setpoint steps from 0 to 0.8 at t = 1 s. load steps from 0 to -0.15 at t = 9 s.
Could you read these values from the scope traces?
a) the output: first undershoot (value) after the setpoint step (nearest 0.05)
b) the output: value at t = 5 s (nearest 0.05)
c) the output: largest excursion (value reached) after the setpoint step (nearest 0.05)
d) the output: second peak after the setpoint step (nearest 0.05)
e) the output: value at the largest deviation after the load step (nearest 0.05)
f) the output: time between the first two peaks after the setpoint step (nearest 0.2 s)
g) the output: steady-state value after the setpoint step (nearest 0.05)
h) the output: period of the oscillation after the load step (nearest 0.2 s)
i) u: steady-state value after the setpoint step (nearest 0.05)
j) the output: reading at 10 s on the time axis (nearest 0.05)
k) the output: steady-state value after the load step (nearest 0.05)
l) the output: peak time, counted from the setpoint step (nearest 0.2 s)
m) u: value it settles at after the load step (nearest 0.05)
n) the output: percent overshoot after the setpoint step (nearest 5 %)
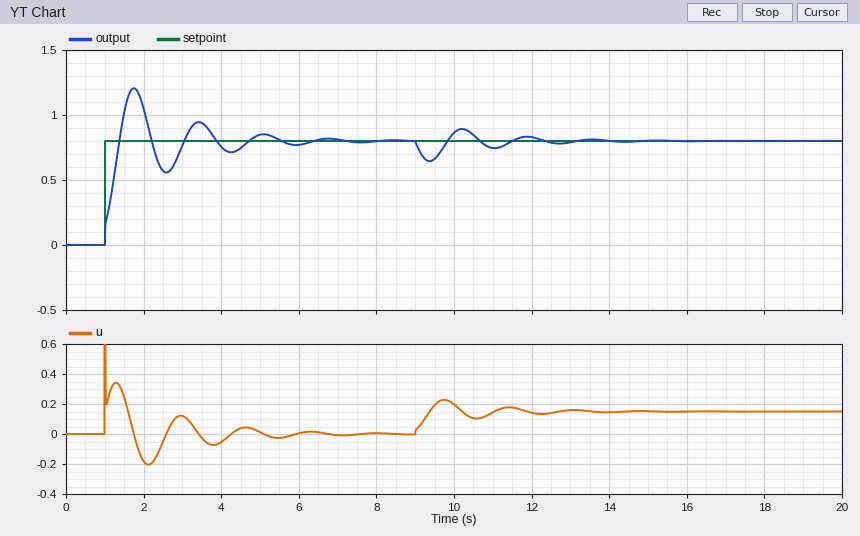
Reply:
0.55
0.85
1.20
0.95
0.65
1.6 s
0.80
1.6 s
0.00
0.85
0.80
0.8 s
0.15
50 %
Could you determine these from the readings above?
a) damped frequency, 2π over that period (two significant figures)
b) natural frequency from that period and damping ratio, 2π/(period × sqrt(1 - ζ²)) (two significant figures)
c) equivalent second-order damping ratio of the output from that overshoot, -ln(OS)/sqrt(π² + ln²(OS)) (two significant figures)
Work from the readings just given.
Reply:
3.9 rad/s
4.0 rad/s
0.22
